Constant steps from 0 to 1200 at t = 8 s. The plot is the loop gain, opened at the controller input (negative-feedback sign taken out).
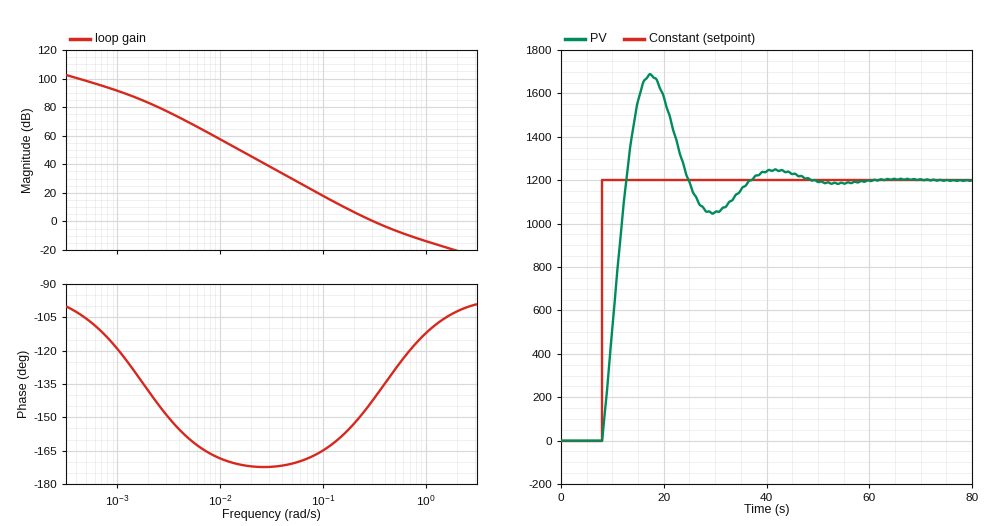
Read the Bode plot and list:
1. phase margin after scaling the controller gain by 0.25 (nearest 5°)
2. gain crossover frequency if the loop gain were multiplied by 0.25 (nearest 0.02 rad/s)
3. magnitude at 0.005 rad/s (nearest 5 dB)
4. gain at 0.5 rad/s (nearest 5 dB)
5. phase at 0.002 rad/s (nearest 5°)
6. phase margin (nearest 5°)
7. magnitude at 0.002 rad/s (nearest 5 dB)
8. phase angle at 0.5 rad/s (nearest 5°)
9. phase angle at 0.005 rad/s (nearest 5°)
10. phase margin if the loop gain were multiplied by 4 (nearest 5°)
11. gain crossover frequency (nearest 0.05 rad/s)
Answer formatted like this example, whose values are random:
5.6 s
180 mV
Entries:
20°
0.14 rad/s
70 dB
-5 dB
-140°
40°
85 dB
-130°
-160°
65°
0.30 rad/s
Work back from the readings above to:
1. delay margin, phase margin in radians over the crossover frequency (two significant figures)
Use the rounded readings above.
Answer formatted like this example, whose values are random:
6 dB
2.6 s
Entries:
2.3 s
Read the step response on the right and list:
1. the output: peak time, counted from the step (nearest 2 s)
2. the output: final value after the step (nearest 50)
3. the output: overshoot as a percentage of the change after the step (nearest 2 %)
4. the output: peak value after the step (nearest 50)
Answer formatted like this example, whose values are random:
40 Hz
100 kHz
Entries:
10 s
1200
40 %
1700
